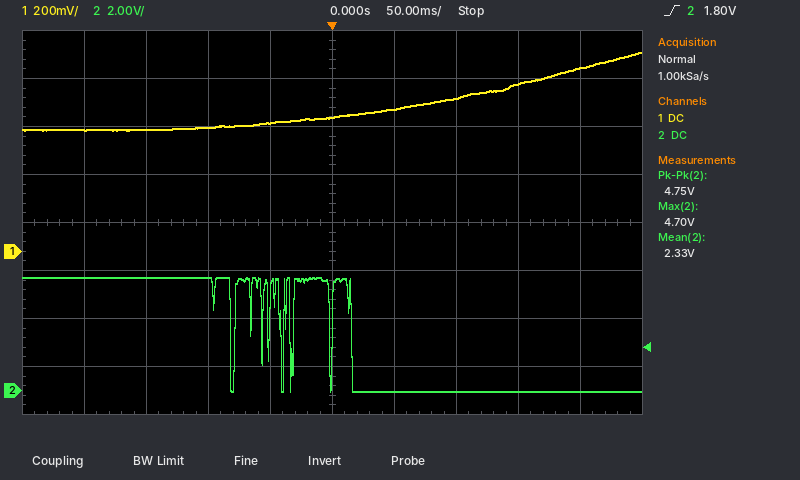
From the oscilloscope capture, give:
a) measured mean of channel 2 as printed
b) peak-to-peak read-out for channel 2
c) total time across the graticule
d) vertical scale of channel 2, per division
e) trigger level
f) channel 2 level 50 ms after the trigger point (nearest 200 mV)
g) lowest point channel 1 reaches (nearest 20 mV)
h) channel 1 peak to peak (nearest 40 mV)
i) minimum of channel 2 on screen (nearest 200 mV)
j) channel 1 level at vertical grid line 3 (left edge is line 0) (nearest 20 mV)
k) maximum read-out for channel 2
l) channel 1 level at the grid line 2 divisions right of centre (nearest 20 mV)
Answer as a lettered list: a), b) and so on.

a) 2.33 V
b) 4.75 V
c) 500 ms
d) 2 V
e) 1.80 V
f) 0.0 V
g) 500 mV
h) 320 mV
i) 0.0 V
j) 520 mV
k) 4.70 V
l) 640 mV
